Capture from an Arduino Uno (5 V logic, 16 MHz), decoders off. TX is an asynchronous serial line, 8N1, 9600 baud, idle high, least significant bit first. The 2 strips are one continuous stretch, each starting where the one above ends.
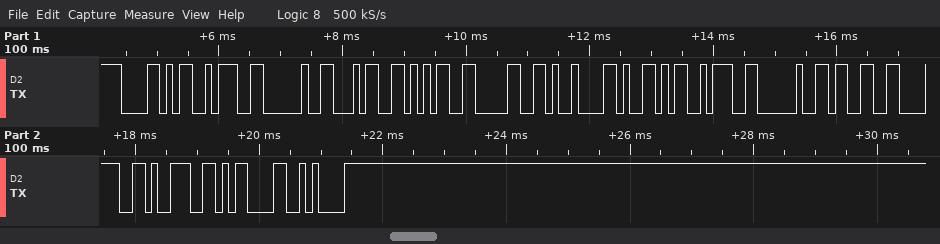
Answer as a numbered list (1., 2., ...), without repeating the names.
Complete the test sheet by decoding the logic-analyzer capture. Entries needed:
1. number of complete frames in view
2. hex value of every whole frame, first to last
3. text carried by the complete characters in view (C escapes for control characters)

1. 15
2. 0x58 0x3A 0x20 0x34 0x35 0x30 0x09 0x59 0x3A 0x20 0x33 0x38 0x39 0x0D 0x0A
3. "X: 450\tY: 389\r\n"
